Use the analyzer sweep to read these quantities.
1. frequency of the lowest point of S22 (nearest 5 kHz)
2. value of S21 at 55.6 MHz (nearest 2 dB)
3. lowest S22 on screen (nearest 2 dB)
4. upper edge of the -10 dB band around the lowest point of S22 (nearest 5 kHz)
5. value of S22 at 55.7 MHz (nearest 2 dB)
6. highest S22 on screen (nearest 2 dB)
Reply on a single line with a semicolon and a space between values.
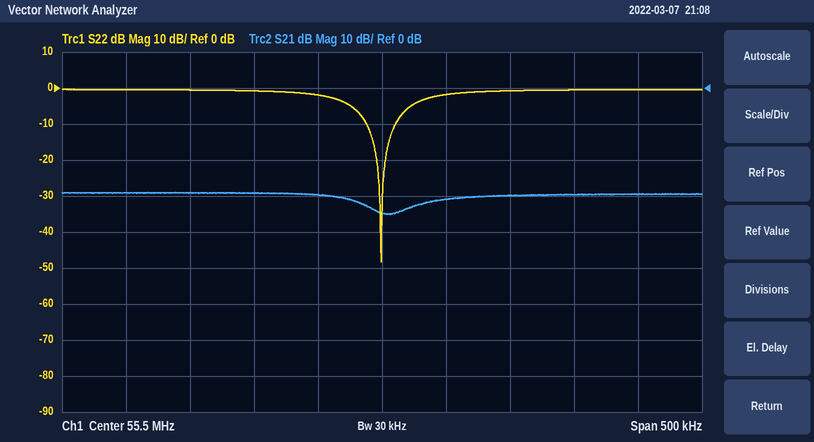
55.500 MHz; -30 dB; -48 dB; 55.510 MHz; 0 dB; 0 dB
